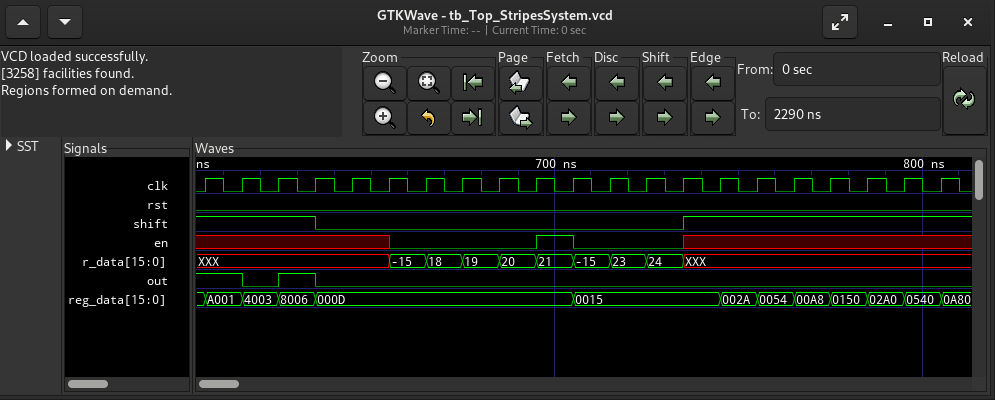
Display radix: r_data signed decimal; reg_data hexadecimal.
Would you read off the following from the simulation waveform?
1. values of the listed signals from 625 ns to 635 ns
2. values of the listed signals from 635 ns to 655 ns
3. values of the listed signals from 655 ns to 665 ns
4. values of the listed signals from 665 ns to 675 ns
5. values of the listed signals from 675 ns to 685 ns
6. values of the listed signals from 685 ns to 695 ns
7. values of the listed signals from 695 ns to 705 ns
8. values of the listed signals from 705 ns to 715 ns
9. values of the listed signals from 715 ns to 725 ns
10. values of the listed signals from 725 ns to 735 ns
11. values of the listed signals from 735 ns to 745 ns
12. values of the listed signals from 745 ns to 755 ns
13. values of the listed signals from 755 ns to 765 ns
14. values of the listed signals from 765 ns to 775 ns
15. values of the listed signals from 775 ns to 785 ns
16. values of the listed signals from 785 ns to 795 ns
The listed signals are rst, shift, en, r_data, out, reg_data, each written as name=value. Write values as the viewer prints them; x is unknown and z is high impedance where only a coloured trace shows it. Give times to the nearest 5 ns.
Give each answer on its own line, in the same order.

rst=0, shift=1, en=x, r_data=XXX, out=1, reg_data=8006
rst=0, shift=0, en=x, r_data=XXX, out=0, reg_data=000D
rst=0, shift=0, en=0, r_data=-15, out=0, reg_data=000D
rst=0, shift=0, en=0, r_data=18, out=0, reg_data=000D
rst=0, shift=0, en=0, r_data=19, out=0, reg_data=000D
rst=0, shift=0, en=0, r_data=20, out=0, reg_data=000D
rst=0, shift=0, en=1, r_data=21, out=0, reg_data=000D
rst=0, shift=0, en=0, r_data=-15, out=0, reg_data=0015
rst=0, shift=0, en=0, r_data=23, out=0, reg_data=0015
rst=0, shift=0, en=0, r_data=24, out=0, reg_data=0015
rst=0, shift=1, en=x, r_data=XXX, out=0, reg_data=0015
rst=0, shift=1, en=x, r_data=XXX, out=0, reg_data=002A
rst=0, shift=1, en=x, r_data=XXX, out=0, reg_data=0054
rst=0, shift=1, en=x, r_data=XXX, out=0, reg_data=00A8
rst=0, shift=1, en=x, r_data=XXX, out=0, reg_data=0150
rst=0, shift=1, en=x, r_data=XXX, out=0, reg_data=02A0
